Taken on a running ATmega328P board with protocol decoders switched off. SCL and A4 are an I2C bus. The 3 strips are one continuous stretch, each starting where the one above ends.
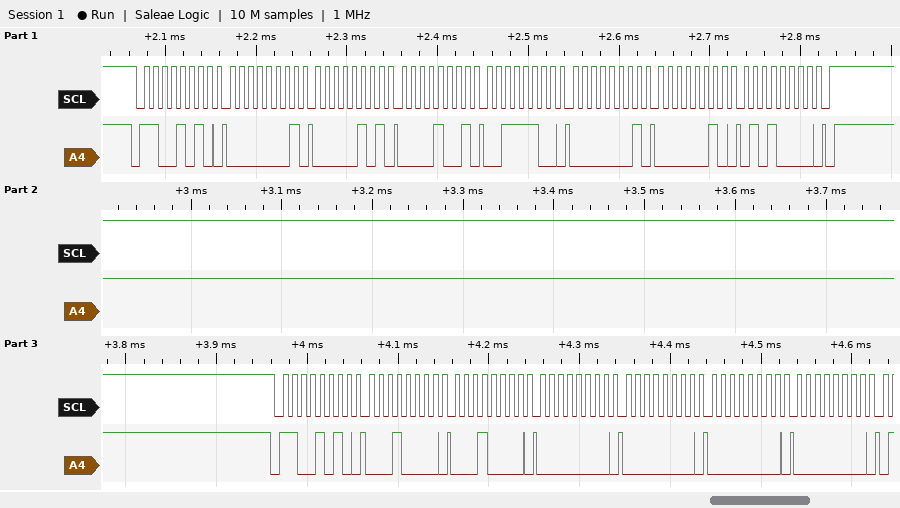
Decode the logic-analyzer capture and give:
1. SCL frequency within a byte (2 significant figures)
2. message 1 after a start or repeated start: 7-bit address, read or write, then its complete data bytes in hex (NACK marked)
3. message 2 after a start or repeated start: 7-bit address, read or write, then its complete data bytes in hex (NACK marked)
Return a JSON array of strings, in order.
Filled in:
["100 kHz", "0x65 write: 01 05 09 3C 01 02 50", "0x65 write: 10 10 00 00 00 00"]
